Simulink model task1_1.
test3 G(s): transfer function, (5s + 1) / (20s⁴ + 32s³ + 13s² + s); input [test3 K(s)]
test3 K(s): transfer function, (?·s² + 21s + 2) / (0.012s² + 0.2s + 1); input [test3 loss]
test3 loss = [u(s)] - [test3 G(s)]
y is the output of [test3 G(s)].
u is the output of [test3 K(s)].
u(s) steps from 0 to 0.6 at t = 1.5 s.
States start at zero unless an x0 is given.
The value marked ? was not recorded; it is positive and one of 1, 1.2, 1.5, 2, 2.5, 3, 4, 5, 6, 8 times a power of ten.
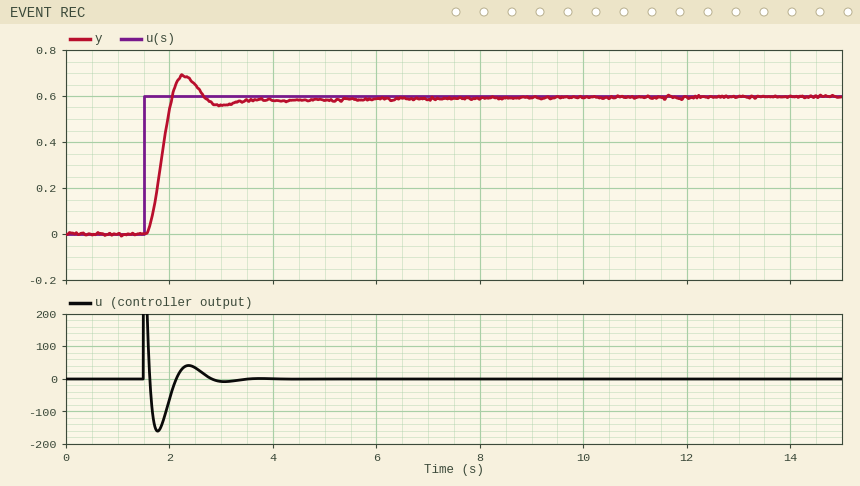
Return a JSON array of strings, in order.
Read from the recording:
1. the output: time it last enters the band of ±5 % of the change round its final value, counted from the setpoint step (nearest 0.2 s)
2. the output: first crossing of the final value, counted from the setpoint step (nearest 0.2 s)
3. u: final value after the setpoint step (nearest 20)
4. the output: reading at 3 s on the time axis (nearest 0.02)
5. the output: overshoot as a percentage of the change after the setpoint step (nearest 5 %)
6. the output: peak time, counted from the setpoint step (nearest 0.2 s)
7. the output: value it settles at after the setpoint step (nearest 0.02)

["1.8 s", "0.6 s", "0", "0.56", "15 %", "0.8 s", "0.60"]
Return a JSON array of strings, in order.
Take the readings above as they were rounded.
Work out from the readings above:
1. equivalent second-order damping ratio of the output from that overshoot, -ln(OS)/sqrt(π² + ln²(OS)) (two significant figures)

["0.52"]
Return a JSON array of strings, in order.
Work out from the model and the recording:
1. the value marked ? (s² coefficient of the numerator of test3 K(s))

["15"]
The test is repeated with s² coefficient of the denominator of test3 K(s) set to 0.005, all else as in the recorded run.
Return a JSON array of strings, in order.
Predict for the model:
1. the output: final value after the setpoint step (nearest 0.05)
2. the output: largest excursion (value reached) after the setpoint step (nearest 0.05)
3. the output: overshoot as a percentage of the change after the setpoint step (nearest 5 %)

["0.60", "0.65", "10 %"]
